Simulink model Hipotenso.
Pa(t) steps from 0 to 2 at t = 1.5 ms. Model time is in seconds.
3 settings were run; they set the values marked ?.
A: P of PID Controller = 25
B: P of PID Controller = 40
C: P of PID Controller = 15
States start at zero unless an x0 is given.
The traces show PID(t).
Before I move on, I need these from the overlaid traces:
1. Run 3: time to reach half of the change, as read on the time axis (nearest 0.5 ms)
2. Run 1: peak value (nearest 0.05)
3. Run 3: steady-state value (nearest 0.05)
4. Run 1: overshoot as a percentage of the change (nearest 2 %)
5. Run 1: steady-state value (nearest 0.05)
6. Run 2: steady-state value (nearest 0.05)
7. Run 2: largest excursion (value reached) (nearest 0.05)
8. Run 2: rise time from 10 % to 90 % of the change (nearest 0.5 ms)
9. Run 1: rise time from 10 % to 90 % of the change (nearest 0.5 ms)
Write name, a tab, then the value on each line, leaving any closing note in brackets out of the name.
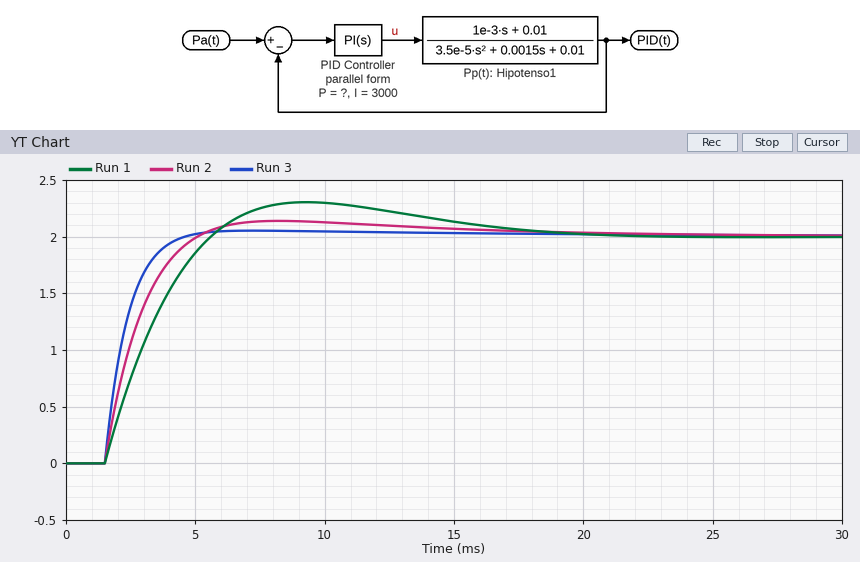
Run 3: time to reach half of the change, as read on the time axis	2.0 ms
Run 1: peak value	2.30
Run 3: steady-state value	2.00
Run 1: overshoot as a percentage of the change	16 %
Run 1: steady-state value	2.00
Run 2: steady-state value	2.00
Run 2: largest excursion (value reached)	2.15
Run 2: rise time from 10 % to 90 % of the change	2.5 ms
Run 1: rise time from 10 % to 90 % of the change	3.0 ms
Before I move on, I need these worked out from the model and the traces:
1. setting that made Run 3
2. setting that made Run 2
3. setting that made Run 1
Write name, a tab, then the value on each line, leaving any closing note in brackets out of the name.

setting that made Run 3	B
setting that made Run 2	A
setting that made Run 1	C
